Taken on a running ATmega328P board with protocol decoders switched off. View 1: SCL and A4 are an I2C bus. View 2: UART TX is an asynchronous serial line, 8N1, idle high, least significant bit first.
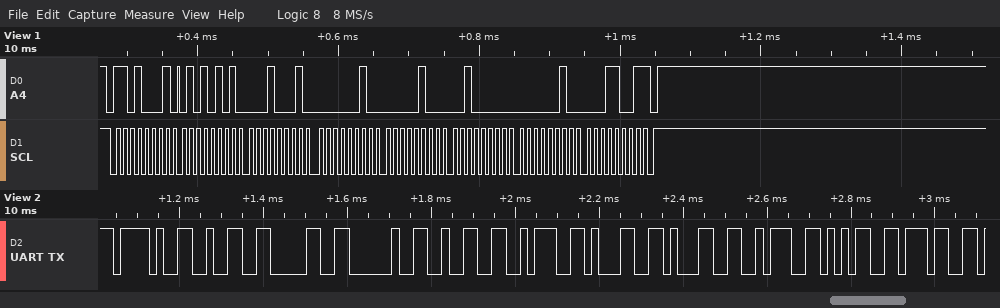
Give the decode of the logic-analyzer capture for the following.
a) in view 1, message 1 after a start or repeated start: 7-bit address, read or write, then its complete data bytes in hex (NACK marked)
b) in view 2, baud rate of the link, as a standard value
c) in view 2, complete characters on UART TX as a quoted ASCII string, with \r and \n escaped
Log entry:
0x68 read: 55 11 02 04 20 02 19 NACK
57600 baud
"/20 2:11:57"
